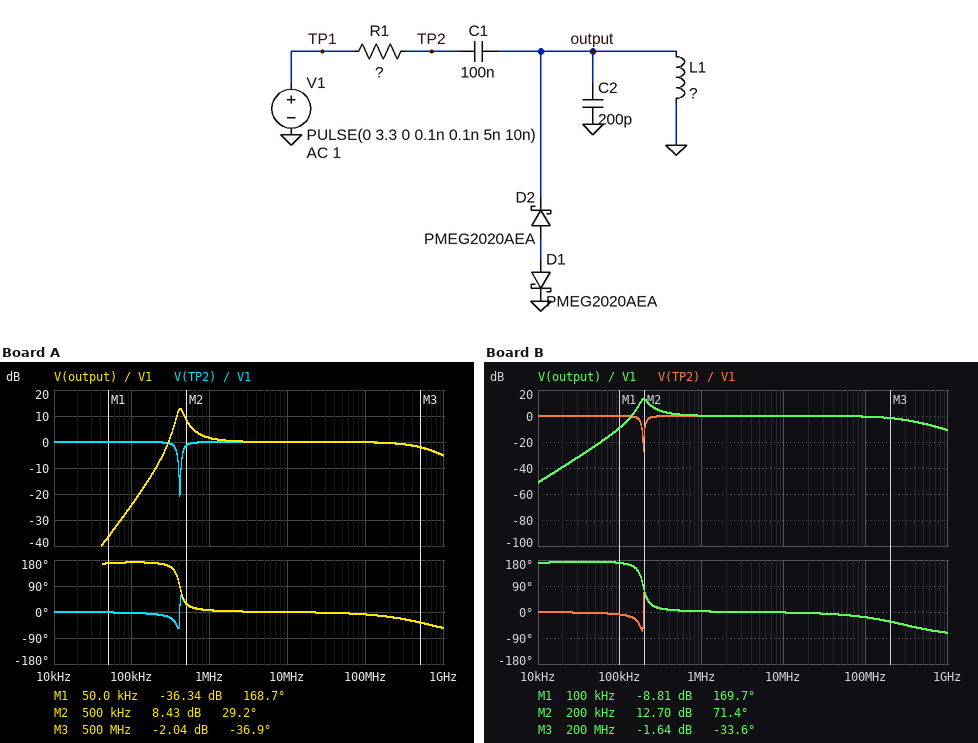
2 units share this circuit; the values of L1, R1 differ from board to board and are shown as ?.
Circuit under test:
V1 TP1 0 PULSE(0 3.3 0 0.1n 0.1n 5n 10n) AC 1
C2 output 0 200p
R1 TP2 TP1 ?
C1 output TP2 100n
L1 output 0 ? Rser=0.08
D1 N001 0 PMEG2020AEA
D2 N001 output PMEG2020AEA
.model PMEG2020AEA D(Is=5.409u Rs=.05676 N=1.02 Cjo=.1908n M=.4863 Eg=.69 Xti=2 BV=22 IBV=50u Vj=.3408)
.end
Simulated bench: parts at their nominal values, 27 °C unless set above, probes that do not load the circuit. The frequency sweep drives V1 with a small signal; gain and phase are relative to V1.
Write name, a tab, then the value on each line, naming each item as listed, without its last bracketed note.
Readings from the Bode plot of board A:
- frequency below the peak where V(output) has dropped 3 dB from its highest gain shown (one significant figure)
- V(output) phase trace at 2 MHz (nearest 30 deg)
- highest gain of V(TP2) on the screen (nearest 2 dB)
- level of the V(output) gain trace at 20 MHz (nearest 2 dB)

frequency below the peak where V(output) has dropped 3 dB from its highest gain shown	400 kHz
V(output) phase trace at 2 MHz	0 deg
highest gain of V(TP2) on the screen	0 dB
level of the V(output) gain trace at 20 MHz	0 dB
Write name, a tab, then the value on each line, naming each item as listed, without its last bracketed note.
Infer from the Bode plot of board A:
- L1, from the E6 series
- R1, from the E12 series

L1, from the E6 series	1.5 µH
R1, from the E12 series	0.82 Ω
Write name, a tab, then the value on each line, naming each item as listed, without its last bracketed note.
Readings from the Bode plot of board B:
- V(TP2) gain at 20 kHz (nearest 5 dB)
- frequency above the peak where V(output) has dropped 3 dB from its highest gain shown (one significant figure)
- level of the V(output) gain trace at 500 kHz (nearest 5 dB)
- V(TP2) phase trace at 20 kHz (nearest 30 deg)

V(TP2) gain at 20 kHz	0 dB
frequency above the peak where V(output) has dropped 3 dB from its highest gain shown	200 kHz
level of the V(output) gain trace at 500 kHz	0 dB
V(TP2) phase trace at 20 kHz	0 deg
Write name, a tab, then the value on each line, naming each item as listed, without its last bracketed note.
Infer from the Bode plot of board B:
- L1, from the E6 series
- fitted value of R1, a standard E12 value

L1, from the E6 series	6.8 µH
fitted value of R1, a standard E12 value	1.8 Ω
